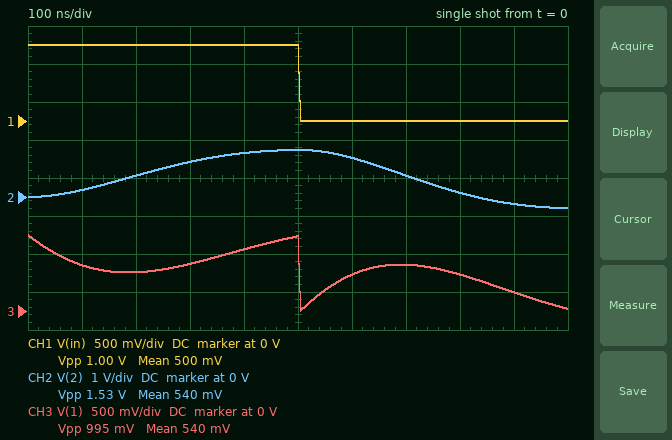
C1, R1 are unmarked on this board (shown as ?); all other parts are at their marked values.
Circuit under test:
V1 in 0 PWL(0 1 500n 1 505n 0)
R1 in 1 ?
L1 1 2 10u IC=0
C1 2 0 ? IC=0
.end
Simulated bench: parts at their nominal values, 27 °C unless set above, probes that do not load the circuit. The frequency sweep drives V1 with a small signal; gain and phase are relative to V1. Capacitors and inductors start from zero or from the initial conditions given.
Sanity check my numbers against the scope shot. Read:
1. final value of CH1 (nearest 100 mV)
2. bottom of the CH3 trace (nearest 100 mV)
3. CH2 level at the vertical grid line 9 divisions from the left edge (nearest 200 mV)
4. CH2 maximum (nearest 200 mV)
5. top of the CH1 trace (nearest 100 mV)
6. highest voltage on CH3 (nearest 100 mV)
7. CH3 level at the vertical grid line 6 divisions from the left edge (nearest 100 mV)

0 V
0 V
-200 mV
1.2 V
1.0 V
1.0 V
500 mV
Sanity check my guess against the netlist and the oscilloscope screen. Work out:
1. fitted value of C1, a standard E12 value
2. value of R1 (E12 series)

2.2 nF
56 Ω
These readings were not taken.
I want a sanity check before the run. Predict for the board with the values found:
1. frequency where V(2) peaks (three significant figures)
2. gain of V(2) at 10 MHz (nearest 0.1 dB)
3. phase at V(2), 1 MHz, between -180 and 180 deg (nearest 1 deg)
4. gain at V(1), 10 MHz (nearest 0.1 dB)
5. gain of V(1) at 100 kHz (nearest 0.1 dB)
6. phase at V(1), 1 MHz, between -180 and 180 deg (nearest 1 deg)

868 kHz
-38.7 dB
-80 deg
0 dB
0 dB
-80 deg
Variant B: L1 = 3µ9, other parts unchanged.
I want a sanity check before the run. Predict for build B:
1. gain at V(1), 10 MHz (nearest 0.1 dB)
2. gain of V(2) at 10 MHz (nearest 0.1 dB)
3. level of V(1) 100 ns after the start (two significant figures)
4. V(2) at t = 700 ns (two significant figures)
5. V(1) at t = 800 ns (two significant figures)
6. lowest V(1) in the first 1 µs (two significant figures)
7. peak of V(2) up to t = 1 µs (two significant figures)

-0.2 dB
-30.6 dB
370 mV
210 mV
140 mV
-40 mV
1.1 V
